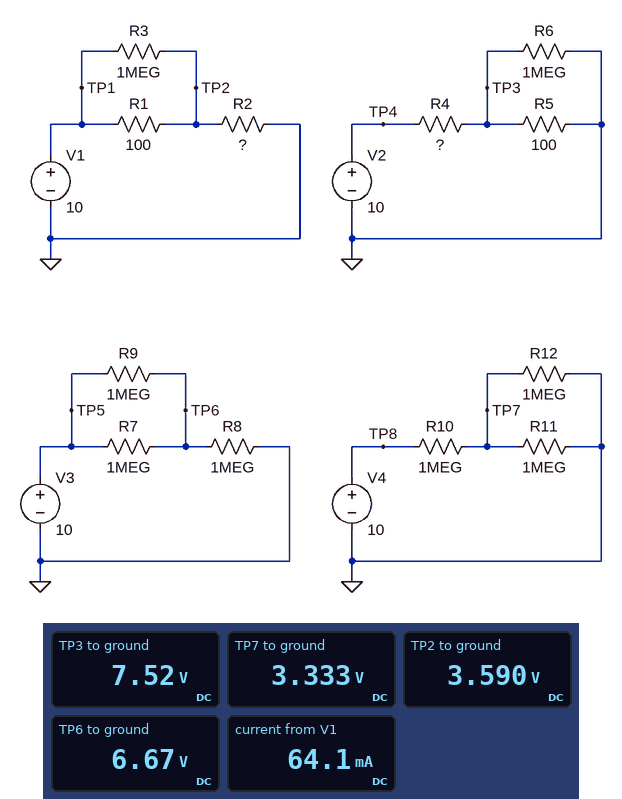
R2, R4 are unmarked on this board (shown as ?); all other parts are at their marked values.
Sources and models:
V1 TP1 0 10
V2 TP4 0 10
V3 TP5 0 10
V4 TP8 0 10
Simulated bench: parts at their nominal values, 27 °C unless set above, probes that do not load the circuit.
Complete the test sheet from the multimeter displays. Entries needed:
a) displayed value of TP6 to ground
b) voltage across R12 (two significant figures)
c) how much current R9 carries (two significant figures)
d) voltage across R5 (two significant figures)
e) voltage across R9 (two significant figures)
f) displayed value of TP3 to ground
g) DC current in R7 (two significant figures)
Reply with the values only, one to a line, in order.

6.67 V
3.3 V
3.3 µA
7.5 V
3.3 V
7.52 V
3.3 µA
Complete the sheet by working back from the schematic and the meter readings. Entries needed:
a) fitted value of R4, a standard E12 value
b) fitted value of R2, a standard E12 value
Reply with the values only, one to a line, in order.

33 Ω
56 Ω
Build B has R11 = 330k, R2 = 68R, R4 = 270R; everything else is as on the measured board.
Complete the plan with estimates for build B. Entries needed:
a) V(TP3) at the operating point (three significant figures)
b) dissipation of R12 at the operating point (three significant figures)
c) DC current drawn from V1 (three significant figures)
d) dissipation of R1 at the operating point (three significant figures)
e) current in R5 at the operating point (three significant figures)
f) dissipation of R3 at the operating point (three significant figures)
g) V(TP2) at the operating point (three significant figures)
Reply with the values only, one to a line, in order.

2.70 V
3.95 µW
59.5 mA
354 mW
27.0 mA
35.4 µW
4.05 V
